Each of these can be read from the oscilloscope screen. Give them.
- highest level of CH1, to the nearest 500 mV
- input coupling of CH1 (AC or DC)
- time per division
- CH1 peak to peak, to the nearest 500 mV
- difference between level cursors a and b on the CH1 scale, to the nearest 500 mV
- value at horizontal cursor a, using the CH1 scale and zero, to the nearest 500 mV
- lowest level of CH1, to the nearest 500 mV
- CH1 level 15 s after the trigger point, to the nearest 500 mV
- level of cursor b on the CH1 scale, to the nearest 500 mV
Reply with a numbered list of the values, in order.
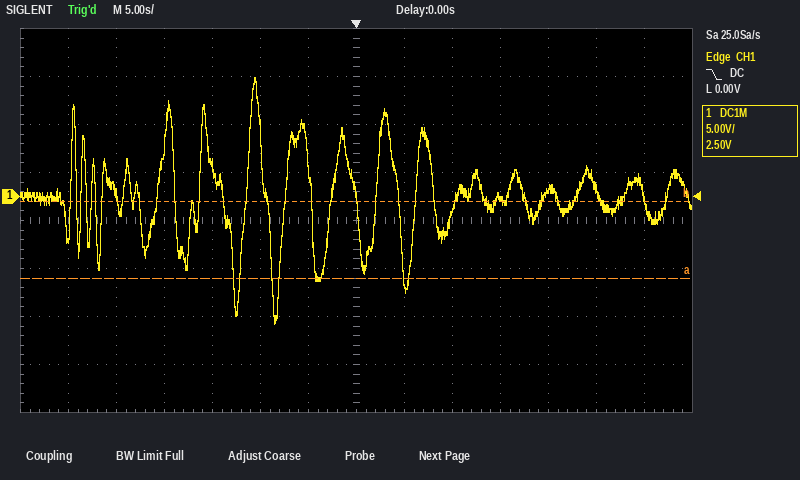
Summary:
1. 12.5 V
2. DC
3. 5 s
4. 25.5 V
5. 8.0 V
6. -8.5 V
7. -13.0 V
8. 0.0 V
9. -500 mV
